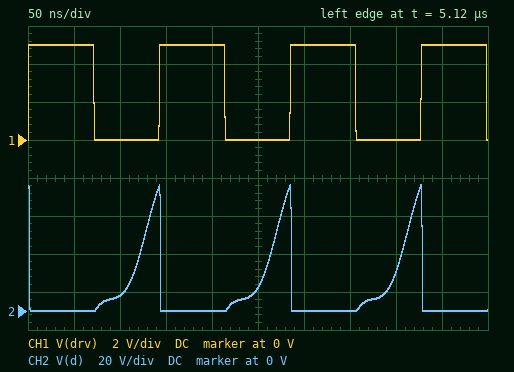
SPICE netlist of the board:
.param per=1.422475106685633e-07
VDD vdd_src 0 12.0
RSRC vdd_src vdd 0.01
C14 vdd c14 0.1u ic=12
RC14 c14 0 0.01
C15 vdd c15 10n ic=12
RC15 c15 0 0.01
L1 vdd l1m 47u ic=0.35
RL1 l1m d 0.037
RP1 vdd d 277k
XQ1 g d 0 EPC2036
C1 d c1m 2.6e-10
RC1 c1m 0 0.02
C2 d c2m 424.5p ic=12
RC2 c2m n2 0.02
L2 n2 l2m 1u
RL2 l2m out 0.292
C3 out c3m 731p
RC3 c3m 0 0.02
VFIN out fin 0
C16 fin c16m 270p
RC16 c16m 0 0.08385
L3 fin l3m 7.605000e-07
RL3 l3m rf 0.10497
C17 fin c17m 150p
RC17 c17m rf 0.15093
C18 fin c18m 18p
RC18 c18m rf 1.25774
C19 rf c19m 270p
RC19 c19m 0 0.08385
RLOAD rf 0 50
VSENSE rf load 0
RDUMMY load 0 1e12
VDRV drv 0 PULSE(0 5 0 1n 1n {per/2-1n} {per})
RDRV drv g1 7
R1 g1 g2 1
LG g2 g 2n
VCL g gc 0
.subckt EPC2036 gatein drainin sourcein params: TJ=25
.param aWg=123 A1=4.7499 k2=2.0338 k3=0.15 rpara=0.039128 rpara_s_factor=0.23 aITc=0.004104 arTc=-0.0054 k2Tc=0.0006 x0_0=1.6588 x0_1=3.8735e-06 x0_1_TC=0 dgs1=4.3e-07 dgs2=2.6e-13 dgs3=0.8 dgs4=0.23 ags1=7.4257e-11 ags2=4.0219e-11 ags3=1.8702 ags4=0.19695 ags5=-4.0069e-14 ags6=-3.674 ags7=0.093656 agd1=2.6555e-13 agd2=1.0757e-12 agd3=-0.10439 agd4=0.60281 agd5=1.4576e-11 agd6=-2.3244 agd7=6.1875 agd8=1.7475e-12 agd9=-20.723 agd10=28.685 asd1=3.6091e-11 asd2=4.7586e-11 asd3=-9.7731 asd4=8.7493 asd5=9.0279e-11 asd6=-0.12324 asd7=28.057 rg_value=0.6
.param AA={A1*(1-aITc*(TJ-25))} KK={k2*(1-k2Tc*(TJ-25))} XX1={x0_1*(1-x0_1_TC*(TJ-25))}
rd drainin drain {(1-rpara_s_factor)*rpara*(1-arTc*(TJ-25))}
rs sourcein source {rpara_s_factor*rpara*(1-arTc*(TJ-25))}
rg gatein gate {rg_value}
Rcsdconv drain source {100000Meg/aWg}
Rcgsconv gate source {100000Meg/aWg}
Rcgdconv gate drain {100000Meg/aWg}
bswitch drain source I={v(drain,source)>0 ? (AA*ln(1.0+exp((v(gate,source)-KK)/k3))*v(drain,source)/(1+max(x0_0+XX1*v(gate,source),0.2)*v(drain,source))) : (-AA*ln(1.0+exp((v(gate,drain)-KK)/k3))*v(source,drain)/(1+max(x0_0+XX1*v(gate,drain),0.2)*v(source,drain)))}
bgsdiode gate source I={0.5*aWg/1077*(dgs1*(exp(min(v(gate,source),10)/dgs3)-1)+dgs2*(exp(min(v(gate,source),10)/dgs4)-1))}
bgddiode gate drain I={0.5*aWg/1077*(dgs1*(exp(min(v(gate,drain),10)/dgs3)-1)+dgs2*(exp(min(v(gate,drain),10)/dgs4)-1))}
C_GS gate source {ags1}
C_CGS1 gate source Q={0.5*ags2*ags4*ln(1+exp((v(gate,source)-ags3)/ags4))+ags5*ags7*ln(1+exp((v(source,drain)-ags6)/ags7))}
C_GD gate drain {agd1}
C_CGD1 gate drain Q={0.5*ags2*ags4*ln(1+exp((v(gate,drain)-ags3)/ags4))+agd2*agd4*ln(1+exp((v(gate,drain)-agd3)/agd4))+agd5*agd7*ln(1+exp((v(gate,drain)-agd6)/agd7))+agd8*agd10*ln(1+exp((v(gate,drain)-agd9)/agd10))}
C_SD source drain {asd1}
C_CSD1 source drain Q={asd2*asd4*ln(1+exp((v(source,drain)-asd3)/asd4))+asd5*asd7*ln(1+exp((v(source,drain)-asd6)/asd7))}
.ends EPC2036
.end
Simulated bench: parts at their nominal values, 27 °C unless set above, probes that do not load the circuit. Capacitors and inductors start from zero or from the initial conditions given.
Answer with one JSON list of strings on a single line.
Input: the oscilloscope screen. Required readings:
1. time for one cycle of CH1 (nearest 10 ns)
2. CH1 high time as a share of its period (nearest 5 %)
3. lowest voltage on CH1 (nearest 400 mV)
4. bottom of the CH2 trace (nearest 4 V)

["140 ns", "50 %", "0 V", "0 V"]
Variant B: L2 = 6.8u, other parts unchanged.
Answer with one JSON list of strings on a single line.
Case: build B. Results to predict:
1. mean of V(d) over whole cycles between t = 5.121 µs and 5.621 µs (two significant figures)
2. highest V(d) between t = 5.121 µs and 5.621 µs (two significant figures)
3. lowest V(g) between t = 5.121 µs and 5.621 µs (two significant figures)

["12 V", "42 V", "1.6 mV"]
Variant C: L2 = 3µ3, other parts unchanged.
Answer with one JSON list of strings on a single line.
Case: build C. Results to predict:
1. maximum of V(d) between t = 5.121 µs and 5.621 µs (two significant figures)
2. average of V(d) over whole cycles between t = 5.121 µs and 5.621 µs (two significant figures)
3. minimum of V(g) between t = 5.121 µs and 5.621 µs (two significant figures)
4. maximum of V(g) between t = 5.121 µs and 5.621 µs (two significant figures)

["34 V", "12 V", "-6.1 mV", "5.0 V"]
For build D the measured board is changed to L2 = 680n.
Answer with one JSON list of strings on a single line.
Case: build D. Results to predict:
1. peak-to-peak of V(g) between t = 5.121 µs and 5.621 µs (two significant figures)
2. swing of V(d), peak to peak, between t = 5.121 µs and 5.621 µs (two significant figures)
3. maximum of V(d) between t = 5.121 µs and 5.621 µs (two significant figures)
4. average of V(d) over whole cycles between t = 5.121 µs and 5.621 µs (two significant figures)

["5.1 V", "65 V", "63 V", "12 V"]
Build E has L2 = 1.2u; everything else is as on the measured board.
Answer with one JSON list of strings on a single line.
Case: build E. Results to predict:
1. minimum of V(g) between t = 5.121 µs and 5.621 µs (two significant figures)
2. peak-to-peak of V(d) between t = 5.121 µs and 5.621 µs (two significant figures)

["3.8 mV", "64 V"]
